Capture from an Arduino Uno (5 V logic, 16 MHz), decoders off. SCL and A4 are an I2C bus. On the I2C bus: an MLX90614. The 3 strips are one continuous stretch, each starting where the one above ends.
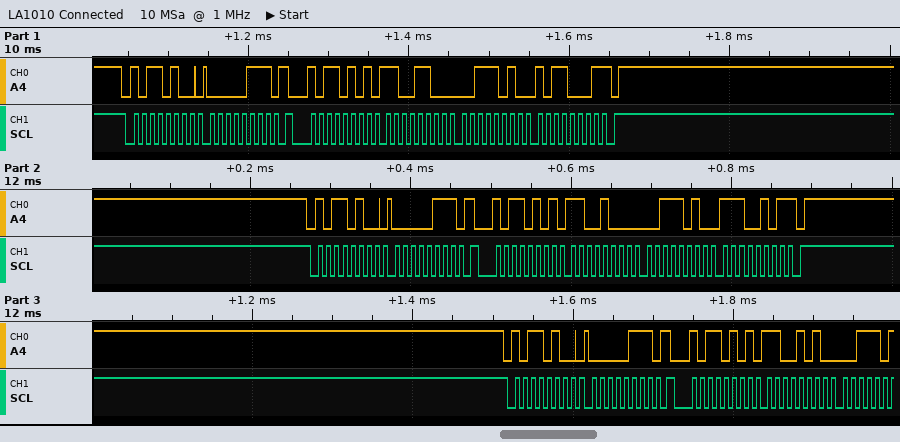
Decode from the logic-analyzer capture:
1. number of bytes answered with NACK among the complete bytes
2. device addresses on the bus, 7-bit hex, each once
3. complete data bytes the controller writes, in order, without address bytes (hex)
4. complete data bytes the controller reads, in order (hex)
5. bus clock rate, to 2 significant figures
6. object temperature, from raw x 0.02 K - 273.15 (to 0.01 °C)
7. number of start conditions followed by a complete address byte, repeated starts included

2
0x5A
07 07 07
CC 3A B1 C8 3A E5 CA
100 kHz
27.89 °C
6
